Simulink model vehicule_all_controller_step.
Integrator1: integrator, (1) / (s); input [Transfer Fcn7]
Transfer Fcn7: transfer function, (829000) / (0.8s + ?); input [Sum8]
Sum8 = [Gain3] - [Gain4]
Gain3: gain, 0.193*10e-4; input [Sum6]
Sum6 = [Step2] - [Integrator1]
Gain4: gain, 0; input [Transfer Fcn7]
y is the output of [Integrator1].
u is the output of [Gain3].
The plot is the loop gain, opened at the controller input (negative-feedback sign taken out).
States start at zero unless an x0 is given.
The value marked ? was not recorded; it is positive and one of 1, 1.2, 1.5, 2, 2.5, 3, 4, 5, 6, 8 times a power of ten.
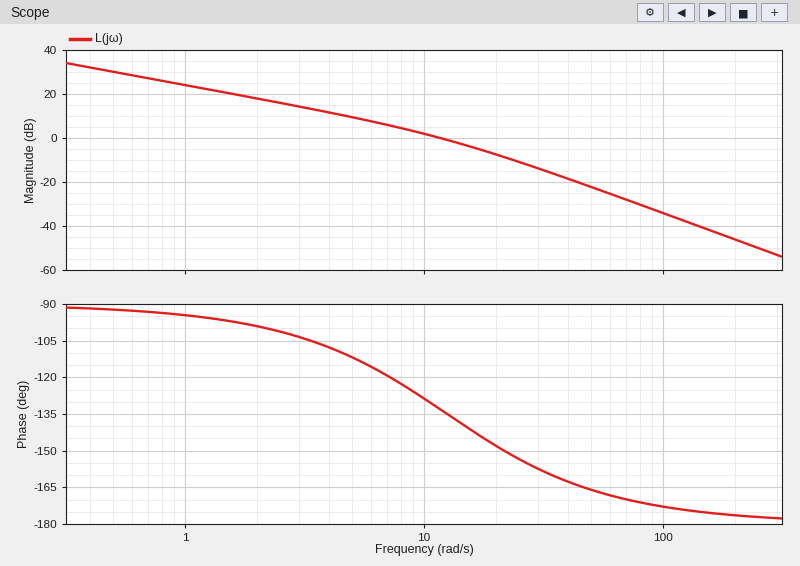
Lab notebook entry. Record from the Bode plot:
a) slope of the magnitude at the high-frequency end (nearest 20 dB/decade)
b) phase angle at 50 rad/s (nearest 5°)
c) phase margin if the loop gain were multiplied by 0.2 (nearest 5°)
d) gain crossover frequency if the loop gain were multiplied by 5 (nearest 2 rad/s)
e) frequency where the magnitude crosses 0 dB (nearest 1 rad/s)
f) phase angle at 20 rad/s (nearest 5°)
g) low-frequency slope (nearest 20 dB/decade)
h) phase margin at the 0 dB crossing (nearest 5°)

-40 dB/decade
-165°
75°
30 rad/s
12 rad/s
-150°
-20 dB/decade
45°
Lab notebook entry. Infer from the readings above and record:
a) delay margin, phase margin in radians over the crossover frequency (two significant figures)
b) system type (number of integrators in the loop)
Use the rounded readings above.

0.065 s
1
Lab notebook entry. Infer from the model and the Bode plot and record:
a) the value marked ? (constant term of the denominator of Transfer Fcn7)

10
